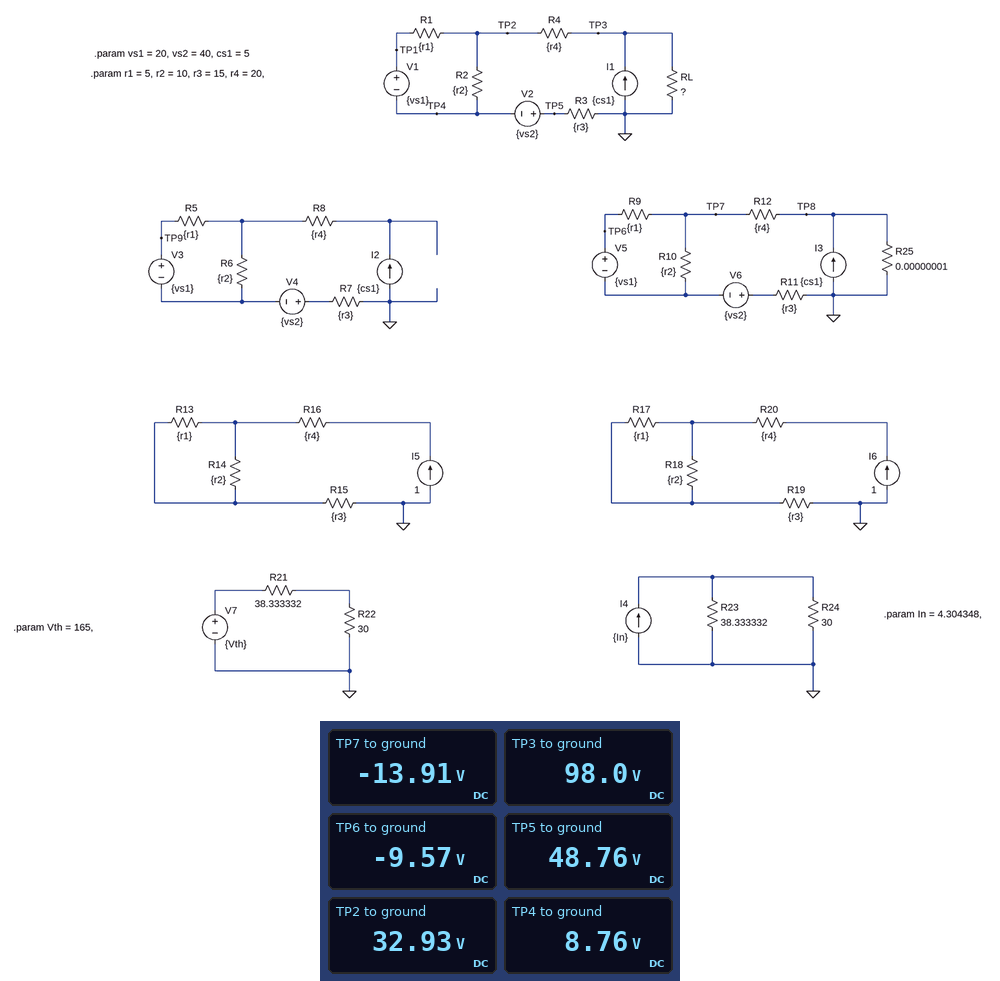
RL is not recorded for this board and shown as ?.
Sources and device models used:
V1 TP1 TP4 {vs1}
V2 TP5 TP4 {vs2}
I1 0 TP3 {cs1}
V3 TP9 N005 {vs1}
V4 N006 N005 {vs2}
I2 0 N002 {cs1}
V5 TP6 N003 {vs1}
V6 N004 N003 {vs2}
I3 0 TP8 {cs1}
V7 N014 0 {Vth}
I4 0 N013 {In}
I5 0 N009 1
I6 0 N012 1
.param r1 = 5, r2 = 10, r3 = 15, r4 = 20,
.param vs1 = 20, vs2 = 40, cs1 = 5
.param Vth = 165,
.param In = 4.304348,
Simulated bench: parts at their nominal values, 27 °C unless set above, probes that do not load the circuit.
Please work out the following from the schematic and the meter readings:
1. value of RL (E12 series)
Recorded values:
56 Ω
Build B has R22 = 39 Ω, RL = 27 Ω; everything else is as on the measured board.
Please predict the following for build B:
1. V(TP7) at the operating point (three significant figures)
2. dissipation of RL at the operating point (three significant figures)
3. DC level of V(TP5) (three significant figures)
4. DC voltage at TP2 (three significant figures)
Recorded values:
-13.9 V
172 W
37.1 V
18.7 V
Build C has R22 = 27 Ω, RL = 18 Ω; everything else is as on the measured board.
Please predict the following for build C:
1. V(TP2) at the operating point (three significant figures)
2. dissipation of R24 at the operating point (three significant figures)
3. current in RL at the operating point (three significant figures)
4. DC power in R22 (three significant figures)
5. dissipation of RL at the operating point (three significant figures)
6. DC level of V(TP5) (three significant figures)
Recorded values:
11.3 V
175 W
2.93 A
172 W
154 W
31.1 V
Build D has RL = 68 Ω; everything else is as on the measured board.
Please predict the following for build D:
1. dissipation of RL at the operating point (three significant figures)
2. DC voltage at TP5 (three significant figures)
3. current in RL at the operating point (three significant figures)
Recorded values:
164 W
51.7 V
1.55 A
